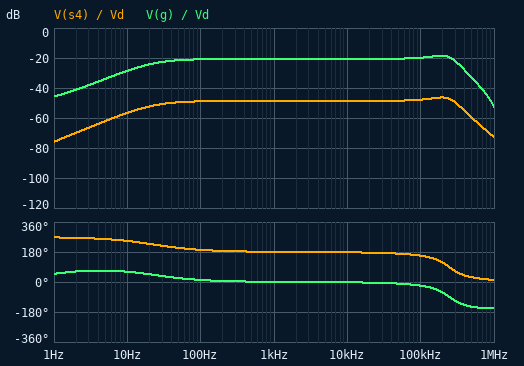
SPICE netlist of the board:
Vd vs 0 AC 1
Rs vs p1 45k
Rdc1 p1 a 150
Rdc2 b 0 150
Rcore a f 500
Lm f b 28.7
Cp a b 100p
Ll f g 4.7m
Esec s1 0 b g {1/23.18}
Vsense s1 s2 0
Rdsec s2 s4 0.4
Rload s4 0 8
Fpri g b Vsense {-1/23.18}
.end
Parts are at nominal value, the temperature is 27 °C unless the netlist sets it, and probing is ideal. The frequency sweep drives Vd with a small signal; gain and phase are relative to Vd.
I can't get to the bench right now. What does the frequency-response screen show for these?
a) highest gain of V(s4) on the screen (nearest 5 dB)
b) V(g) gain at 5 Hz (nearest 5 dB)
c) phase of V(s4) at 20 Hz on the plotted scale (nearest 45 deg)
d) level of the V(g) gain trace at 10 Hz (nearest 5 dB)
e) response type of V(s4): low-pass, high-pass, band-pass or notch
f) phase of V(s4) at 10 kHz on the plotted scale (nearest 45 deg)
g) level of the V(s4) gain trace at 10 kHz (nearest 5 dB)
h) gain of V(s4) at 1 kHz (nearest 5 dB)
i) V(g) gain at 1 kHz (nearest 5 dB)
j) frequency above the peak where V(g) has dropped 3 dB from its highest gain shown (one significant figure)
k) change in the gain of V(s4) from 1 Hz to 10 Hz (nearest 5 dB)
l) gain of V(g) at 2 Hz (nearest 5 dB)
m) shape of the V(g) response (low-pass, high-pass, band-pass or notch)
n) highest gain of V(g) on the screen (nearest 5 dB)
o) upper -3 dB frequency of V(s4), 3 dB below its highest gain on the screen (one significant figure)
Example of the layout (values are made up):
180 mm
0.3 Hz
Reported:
-45 dB
-35 dB
225 deg
-30 dB
band-pass
180 deg
-50 dB
-50 dB
-20 dB
300 kHz
20 dB
-40 dB
band-pass
-20 dB
300 kHz
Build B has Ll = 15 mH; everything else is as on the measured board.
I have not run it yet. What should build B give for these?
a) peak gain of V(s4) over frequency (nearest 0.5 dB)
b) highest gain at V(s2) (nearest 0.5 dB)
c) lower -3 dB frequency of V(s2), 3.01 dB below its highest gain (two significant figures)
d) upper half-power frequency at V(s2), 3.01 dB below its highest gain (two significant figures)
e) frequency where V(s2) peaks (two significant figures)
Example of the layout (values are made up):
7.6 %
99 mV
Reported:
-44.5 dB
-44.0 dB
58 kHz
160 kHz
120 kHz
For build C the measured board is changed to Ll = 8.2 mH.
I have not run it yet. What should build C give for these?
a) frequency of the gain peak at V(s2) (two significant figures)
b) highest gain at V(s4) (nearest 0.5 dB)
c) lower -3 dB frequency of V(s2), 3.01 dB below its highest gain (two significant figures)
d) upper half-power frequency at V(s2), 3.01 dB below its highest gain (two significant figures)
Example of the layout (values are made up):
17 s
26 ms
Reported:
160 kHz
-45.0 dB
51 kHz
220 kHz
